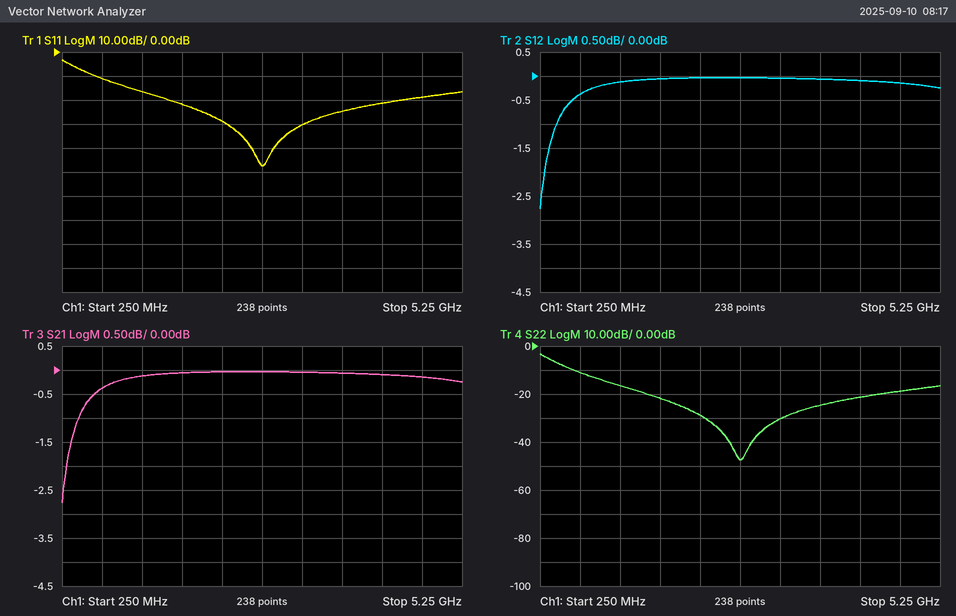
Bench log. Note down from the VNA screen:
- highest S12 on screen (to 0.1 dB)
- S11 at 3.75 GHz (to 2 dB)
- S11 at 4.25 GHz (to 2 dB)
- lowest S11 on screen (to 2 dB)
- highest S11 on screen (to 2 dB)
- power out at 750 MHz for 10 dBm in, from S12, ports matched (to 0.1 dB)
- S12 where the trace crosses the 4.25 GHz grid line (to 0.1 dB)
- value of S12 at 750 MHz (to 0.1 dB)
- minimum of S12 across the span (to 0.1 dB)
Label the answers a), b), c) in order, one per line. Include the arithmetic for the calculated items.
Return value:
a) 0.0 dB
b) -24 dB
c) -22 dB
d) -48 dB
e) -4 dB
f) 10 dBm + (-0.4 dB) = 9.6 dBm
g) -0.1 dB
h) -0.4 dB
i) -2.8 dB
